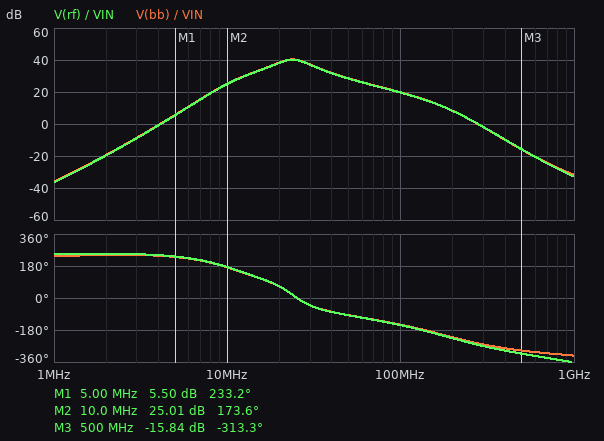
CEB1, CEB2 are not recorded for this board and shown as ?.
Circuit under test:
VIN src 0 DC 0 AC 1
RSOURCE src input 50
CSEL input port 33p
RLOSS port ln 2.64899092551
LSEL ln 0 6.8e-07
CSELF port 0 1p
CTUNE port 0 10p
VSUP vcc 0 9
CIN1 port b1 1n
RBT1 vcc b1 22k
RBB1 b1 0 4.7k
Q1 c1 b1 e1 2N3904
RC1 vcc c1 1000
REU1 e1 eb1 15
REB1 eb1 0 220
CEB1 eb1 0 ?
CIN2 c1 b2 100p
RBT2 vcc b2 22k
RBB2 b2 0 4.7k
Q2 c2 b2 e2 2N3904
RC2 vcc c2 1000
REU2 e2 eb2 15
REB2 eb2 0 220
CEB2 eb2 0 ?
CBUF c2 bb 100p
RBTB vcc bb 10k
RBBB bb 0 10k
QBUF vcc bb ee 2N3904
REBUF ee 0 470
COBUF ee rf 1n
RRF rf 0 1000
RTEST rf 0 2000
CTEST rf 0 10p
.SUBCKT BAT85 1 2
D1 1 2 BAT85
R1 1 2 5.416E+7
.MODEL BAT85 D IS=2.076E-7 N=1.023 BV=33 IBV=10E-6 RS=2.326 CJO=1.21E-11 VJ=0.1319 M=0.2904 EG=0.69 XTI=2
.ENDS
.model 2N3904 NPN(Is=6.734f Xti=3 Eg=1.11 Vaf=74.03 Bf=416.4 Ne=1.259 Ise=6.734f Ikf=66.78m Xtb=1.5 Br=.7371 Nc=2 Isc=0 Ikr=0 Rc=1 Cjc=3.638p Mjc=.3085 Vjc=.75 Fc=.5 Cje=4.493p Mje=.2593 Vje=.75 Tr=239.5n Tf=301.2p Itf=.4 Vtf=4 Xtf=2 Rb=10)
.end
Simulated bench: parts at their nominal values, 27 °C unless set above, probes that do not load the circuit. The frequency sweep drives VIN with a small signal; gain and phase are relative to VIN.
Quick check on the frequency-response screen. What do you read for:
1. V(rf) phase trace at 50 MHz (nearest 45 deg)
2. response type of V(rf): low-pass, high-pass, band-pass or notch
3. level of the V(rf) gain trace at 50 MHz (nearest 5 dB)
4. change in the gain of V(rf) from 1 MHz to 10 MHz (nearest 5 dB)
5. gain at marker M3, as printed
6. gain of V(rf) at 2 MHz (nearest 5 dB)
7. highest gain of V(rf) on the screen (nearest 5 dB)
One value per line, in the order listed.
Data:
-90 deg
band-pass
30 dB
60 dB
-15.84 dB
-20 dB
40 dB
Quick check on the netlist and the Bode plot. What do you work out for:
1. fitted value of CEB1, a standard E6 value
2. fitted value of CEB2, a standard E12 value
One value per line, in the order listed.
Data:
1 nF
150 pF
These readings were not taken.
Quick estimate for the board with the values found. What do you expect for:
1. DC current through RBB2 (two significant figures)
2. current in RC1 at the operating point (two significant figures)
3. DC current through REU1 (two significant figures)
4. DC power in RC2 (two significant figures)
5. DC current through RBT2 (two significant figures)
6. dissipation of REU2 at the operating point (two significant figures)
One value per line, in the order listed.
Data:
320 µA
3.4 mA
3.4 mA
12 mW
340 µA
180 µW
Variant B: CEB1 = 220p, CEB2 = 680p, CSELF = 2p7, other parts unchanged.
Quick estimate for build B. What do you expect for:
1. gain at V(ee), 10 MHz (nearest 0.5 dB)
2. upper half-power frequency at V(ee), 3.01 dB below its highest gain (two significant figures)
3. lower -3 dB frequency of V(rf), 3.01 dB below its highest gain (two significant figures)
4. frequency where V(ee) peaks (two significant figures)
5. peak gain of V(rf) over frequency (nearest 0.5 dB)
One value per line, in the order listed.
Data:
17.5 dB
27 MHz
23 MHz
25 MHz
45.0 dB
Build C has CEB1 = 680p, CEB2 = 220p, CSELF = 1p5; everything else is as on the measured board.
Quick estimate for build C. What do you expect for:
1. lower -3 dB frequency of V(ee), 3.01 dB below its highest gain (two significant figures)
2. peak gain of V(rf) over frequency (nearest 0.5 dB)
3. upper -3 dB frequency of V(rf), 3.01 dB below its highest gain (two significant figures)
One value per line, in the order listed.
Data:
20 MHz
42.0 dB
28 MHz
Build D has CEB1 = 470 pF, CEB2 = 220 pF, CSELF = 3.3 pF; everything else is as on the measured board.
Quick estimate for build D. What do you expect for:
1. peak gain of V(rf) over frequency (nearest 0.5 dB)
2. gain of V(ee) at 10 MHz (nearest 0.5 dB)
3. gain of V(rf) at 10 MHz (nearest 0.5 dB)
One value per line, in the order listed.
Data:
42.5 dB
23.0 dB
22.5 dB
